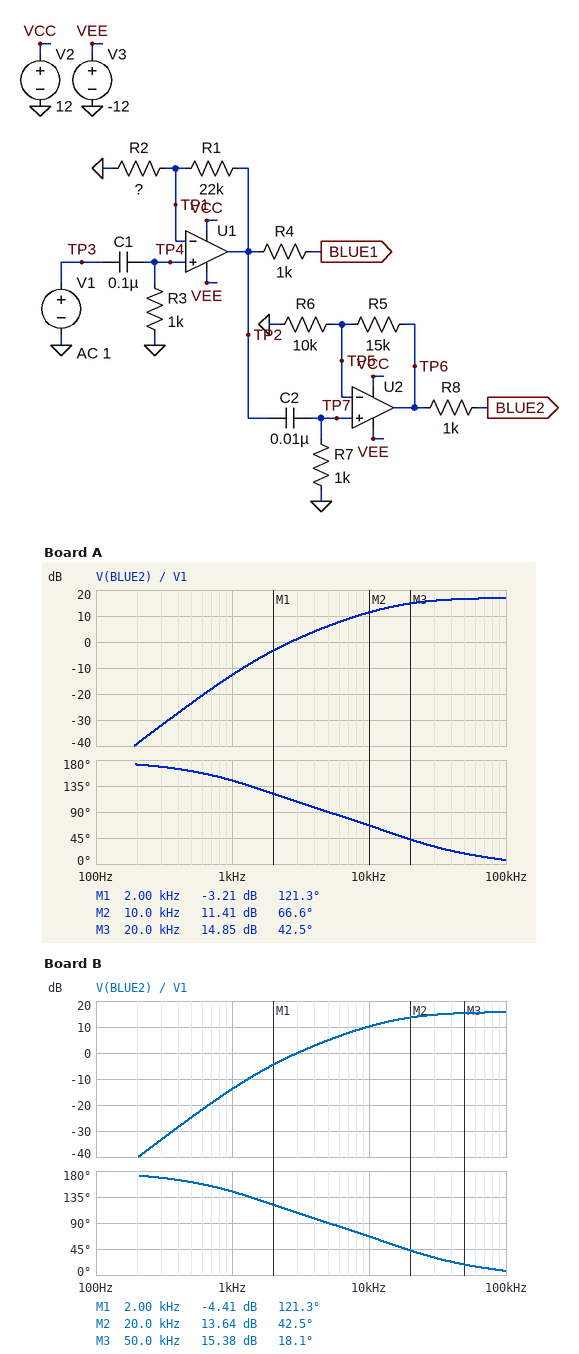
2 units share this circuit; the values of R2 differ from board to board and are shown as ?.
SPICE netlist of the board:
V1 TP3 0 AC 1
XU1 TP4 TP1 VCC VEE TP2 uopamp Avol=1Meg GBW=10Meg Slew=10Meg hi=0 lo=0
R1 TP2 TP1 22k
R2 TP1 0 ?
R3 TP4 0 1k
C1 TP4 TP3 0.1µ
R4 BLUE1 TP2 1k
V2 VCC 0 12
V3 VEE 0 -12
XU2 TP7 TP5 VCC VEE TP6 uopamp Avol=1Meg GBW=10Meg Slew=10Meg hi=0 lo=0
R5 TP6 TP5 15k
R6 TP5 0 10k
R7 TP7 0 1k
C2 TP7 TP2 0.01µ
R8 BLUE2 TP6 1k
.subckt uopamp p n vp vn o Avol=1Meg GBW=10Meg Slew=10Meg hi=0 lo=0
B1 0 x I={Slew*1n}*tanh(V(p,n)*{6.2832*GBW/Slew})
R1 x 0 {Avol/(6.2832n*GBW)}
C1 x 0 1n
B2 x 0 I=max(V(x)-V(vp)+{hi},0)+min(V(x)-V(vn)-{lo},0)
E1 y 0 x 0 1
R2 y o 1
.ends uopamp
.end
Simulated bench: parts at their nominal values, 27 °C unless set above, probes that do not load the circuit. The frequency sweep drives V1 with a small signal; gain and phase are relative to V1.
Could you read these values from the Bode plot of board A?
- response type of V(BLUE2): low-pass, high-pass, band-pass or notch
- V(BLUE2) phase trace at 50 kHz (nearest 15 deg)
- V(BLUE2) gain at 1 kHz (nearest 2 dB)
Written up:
high-pass
15 deg
-12 dB
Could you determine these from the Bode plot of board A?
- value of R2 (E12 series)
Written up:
12 kΩ
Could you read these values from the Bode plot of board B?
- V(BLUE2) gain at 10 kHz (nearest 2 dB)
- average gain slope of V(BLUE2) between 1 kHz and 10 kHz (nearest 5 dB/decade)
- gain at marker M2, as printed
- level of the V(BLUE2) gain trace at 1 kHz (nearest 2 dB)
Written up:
10 dB
25 dB/decade
13.64 dB
-14 dB
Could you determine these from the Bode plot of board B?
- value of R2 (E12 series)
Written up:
15 kΩ
